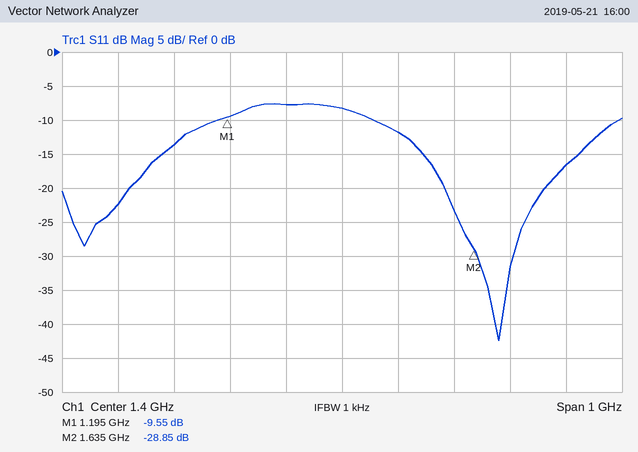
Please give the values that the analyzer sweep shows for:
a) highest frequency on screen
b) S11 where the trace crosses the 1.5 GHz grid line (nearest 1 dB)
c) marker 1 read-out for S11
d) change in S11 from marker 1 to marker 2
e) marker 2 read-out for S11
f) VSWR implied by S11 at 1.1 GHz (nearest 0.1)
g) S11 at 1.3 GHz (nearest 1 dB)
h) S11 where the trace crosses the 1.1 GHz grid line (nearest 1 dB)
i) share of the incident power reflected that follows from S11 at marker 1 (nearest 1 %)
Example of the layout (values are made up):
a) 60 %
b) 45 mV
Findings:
a) 1.9 GHz
b) -12 dB
c) -9.55 dB
d) -19.30 dB
e) -28.85 dB
f) 1.5
g) -8 dB
h) -14 dB
i) 11 %
